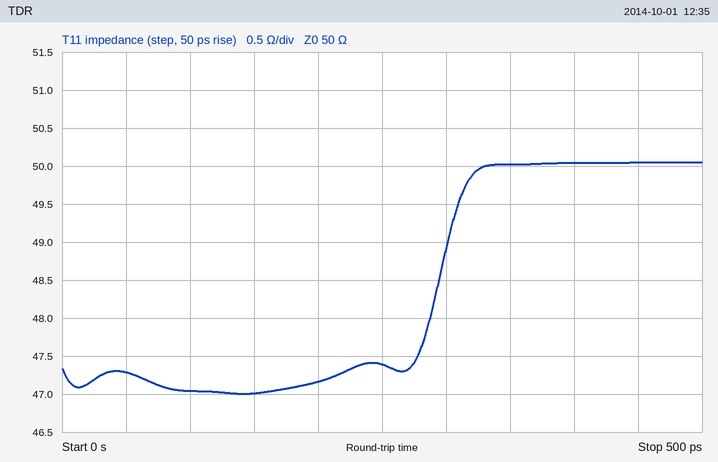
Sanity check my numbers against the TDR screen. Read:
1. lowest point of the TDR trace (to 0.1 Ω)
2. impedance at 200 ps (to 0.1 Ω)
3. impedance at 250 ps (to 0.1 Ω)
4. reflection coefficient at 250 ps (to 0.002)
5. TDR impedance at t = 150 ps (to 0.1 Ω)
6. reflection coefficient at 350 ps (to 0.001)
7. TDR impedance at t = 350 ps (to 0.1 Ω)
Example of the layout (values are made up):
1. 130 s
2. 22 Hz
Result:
1. 47.0 Ω
2. 47.2 Ω
3. 47.4 Ω
4. -0.026
5. 47.0 Ω
6. 0.000
7. 50.0 Ω
